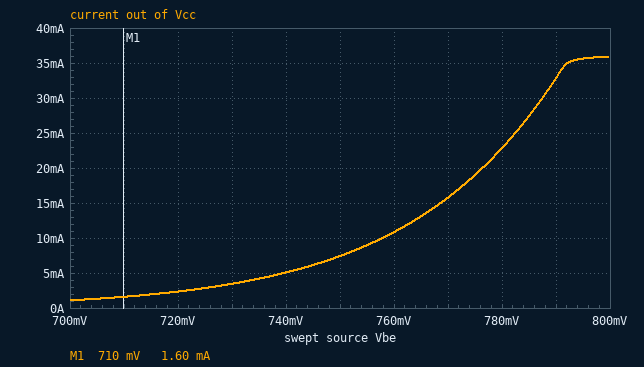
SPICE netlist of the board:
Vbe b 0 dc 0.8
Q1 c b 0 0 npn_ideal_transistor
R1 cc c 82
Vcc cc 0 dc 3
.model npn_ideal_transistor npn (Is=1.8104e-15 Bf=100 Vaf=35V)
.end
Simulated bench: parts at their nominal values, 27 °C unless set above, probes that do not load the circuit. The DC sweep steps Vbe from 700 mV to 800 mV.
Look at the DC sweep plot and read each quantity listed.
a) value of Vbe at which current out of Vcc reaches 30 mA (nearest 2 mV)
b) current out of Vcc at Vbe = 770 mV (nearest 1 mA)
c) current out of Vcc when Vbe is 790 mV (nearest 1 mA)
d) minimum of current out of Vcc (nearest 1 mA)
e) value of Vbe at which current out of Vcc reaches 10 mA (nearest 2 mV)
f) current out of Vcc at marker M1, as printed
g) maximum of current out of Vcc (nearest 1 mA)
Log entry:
788 mV
16 mA
33 mA
1 mA
758 mV
1.60 mA
36 mA
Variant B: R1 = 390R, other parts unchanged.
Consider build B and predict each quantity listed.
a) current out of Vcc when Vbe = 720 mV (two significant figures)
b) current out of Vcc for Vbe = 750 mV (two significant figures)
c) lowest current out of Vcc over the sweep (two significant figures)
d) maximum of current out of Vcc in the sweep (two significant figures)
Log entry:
2.3 mA
7.0 mA
1.1 mA
7.6 mA
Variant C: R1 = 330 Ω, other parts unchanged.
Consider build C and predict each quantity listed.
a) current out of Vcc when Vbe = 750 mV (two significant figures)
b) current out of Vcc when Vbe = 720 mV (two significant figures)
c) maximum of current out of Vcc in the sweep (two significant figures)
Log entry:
7.1 mA
2.3 mA
9.0 mA
